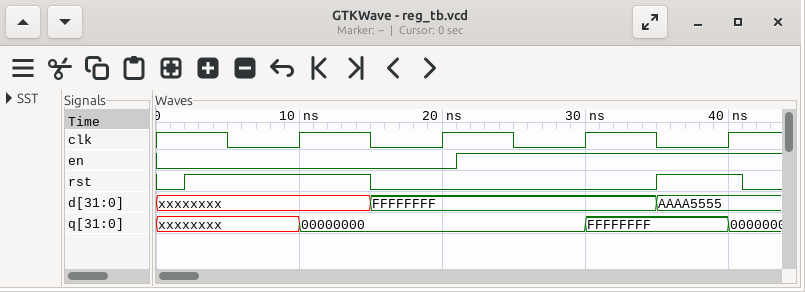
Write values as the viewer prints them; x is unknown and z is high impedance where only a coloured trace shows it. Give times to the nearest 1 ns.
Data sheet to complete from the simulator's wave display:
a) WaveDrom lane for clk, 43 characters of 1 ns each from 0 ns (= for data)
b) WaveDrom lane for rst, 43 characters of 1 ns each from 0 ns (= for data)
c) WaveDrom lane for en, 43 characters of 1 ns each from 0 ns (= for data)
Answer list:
{name: 'clk', wave: '1....0....1....0....1....0....1....0....1..'}
{name: 'rst', wave: '0.1............0...................1.....0.'}
{name: 'en', wave: '0....................1.....................'}
